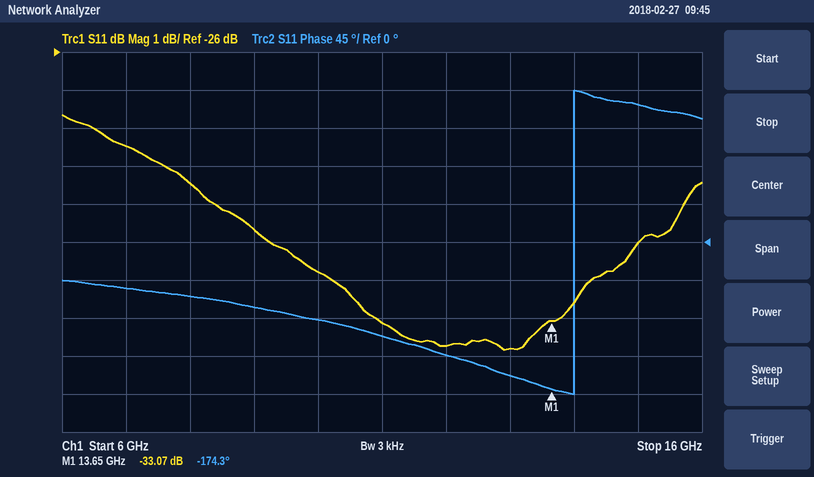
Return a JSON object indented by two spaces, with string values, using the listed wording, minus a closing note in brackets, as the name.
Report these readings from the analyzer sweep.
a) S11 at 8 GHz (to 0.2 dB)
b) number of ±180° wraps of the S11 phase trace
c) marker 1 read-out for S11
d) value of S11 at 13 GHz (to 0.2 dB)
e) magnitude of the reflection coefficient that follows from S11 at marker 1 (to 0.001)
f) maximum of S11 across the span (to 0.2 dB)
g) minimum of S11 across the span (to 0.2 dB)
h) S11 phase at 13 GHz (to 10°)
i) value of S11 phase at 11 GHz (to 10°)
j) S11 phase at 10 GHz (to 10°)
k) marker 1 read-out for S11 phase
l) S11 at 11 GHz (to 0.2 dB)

{
  "S11 at 8 GHz": "-29.4 dB",
  "number of ±180° wraps of the S11 phase trace": "1",
  "marker 1 read-out for S11": "-33.07 dB",
  "value of S11 at 13 GHz": "-33.8 dB",
  "magnitude of the reflection coefficient that follows from S11 at marker 1": "0.022",
  "maximum of S11 across the span": "-27.6 dB",
  "minimum of S11 across the span": "-33.8 dB",
  "S11 phase at 13 GHz": "-160°",
  "value of S11 phase at 11 GHz": "-110°",
  "S11 phase at 10 GHz": "-90°",
  "marker 1 read-out for S11 phase": "-174.3°",
  "S11 at 11 GHz": "-33.2 dB"
}
